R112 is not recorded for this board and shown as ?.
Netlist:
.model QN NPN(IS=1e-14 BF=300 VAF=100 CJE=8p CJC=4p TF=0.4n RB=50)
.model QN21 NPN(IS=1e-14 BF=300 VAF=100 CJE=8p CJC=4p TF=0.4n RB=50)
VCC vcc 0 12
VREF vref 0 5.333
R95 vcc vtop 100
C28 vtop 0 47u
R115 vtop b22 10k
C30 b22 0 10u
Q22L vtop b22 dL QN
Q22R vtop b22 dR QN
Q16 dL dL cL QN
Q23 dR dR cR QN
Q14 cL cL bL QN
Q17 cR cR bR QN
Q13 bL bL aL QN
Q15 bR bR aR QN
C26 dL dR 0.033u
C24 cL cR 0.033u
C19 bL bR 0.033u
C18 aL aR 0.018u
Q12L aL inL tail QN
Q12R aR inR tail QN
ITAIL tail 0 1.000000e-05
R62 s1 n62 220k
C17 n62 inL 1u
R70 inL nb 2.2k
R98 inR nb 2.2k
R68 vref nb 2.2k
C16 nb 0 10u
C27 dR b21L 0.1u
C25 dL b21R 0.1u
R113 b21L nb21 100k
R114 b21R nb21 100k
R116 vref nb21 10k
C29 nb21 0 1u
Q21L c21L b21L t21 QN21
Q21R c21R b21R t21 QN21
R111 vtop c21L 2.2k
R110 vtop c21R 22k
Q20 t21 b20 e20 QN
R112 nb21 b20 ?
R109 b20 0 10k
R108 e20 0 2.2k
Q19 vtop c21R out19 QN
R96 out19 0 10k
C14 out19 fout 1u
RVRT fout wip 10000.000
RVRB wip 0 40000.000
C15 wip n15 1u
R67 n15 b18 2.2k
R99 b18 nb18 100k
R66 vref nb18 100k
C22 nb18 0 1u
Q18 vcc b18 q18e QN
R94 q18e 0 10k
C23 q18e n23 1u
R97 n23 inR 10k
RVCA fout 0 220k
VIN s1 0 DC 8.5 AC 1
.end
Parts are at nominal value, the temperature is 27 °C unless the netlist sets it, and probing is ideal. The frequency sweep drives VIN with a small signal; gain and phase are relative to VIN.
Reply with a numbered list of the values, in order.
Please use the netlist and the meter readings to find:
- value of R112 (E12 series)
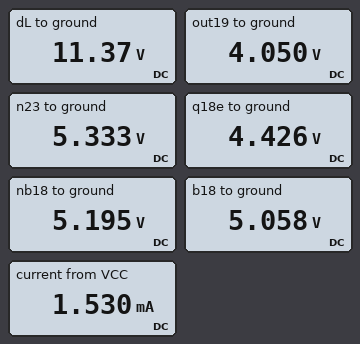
1. 4.7 kΩ
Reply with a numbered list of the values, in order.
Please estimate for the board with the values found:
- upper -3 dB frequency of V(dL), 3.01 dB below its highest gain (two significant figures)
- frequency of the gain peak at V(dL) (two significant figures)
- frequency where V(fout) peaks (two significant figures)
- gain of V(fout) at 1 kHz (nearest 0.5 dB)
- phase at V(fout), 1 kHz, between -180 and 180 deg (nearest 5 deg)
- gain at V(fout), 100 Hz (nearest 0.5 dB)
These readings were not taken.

1. 10 Hz
2. 8.8 Hz
3. 9.0 Hz
4. -27.5 dB
5. 140 deg
6. -23.5 dB
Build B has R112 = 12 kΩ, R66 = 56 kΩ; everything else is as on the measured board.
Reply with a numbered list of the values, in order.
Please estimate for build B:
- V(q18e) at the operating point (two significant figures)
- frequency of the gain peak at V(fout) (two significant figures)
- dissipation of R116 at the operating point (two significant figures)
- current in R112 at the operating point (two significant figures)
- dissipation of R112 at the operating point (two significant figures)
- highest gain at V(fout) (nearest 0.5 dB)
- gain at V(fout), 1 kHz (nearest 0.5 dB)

1. 4.5 V
2. 9.2 Hz
3. 280 µW
4. 170 µA
5. 330 µW
6. -9.5 dB
7. -31.5 dB
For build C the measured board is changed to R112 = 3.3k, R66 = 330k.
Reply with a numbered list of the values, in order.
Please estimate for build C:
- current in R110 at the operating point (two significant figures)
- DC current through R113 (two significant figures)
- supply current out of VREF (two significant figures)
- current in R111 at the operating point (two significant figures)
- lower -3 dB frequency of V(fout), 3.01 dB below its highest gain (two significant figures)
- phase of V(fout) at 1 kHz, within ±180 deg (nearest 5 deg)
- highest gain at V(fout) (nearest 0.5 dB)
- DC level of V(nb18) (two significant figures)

1. 350 µA
2. 1.2 µA
3. 230 µA
4. 380 µA
5. 7.9 Hz
6. 140 deg
7. -7.5 dB
8. 4.9 V
